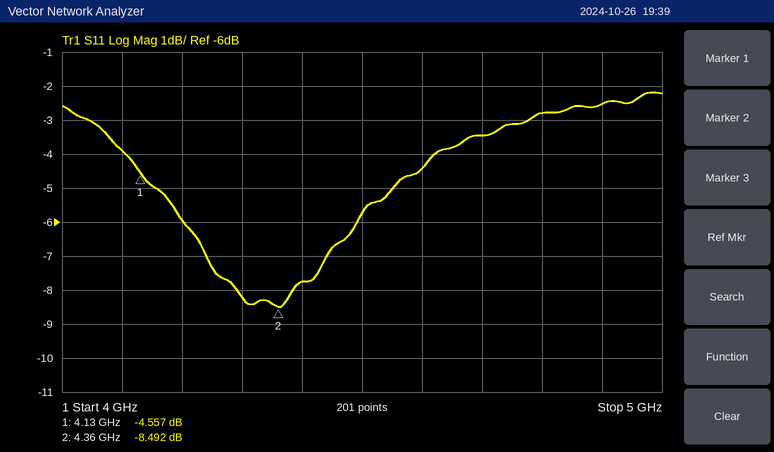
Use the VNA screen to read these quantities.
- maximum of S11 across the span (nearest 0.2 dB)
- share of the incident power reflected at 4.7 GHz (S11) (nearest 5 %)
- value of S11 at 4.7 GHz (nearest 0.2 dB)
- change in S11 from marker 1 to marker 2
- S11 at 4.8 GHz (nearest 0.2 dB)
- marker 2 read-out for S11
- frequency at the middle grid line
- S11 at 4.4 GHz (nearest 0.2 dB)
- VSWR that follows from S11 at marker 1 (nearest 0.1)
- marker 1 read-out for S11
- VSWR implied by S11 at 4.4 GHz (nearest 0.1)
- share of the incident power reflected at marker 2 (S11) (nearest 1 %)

-2.2 dB
45 %
-3.4 dB
-3.935 dB
-2.8 dB
-8.492 dB
4.5 GHz
-7.8 dB
3.9
-4.557 dB
2.4
14 %
